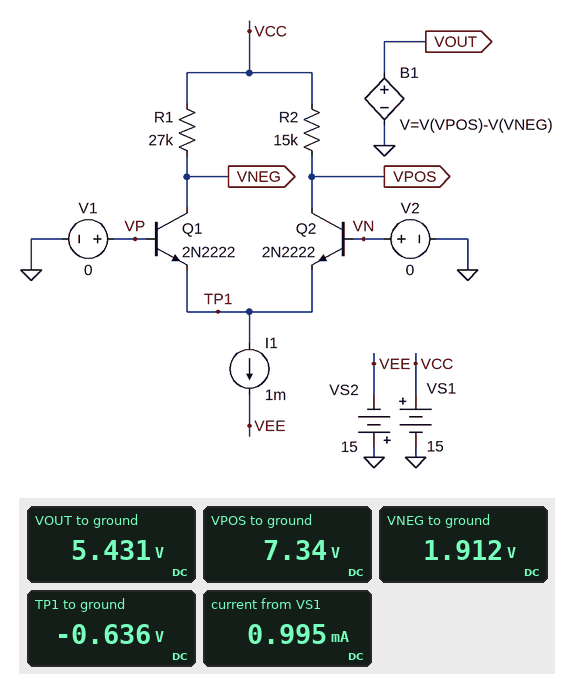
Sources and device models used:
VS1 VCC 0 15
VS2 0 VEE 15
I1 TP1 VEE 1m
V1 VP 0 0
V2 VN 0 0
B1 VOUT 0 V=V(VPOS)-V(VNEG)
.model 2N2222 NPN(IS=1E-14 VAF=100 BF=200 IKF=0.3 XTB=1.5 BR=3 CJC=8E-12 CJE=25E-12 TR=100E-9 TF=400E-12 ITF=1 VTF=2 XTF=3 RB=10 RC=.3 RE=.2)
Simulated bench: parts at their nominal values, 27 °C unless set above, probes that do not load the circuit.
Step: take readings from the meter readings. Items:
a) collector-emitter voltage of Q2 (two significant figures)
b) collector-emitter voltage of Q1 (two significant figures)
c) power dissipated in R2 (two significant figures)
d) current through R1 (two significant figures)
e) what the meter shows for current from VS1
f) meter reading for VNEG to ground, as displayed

8.0 V
2.5 V
3.9 mW
480 µA
0.995 mA
1.912 V
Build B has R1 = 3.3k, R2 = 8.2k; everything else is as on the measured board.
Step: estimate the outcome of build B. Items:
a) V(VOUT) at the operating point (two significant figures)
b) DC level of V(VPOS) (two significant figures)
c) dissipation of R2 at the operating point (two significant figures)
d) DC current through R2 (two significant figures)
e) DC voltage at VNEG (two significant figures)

-2.4 V
11 V
2.0 mW
490 µA
13 V
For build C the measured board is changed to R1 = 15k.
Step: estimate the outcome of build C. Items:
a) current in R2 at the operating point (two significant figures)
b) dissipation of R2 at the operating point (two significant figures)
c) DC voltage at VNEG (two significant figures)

500 µA
3.7 mW
7.5 V
